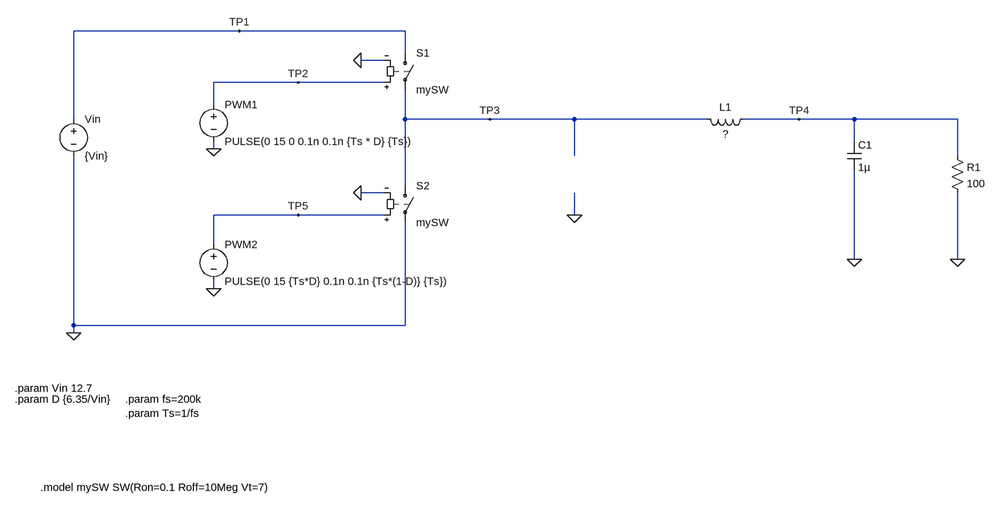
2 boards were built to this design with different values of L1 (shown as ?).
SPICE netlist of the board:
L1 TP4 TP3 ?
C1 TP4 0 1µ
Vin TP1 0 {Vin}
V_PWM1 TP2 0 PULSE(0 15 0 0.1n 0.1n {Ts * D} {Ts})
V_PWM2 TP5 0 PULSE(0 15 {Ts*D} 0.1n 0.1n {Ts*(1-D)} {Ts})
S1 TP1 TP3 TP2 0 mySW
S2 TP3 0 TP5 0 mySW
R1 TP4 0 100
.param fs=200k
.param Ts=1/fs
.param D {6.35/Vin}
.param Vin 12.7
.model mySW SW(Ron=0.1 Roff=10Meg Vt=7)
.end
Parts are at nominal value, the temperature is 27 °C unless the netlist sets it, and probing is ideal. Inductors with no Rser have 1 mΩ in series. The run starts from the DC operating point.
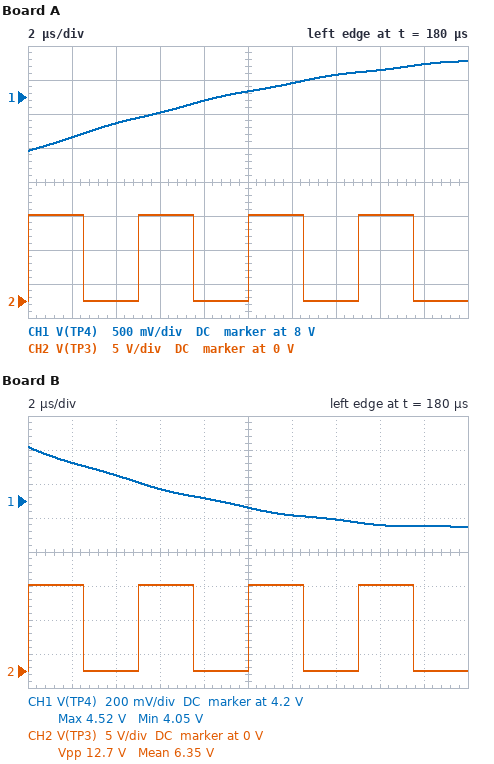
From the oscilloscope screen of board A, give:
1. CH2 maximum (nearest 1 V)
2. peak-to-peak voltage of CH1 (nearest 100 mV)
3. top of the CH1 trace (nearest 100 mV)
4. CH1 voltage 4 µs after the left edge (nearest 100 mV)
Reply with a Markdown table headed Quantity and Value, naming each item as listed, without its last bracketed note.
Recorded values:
| Quantity | Value |
|---|---|
| CH2 maximum | 13 V |
| peak-to-peak voltage of CH1 | 1.3 V |
| top of the CH1 trace | 8.5 V |
| CH1 voltage 4 µs after the left edge | 7.6 V |
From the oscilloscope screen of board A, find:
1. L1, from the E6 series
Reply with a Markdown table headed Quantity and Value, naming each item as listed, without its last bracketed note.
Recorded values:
| Quantity | Value |
|---|---|
| L1, from the E6 series | 470 µH |
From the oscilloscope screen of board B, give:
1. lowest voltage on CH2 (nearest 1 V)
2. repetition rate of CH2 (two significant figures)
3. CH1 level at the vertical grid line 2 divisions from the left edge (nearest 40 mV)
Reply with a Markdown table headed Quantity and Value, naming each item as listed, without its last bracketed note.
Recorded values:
| Quantity | Value |
|---|---|
| lowest voltage on CH2 | 0 V |
| repetition rate of CH2 | 200 kHz |
| CH1 level at the vertical grid line 2 divisions from the left edge | 4.36 V |
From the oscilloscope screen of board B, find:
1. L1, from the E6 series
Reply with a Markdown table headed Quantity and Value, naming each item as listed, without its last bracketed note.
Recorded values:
| Quantity | Value |
|---|---|
| L1, from the E6 series | 1 mH |
